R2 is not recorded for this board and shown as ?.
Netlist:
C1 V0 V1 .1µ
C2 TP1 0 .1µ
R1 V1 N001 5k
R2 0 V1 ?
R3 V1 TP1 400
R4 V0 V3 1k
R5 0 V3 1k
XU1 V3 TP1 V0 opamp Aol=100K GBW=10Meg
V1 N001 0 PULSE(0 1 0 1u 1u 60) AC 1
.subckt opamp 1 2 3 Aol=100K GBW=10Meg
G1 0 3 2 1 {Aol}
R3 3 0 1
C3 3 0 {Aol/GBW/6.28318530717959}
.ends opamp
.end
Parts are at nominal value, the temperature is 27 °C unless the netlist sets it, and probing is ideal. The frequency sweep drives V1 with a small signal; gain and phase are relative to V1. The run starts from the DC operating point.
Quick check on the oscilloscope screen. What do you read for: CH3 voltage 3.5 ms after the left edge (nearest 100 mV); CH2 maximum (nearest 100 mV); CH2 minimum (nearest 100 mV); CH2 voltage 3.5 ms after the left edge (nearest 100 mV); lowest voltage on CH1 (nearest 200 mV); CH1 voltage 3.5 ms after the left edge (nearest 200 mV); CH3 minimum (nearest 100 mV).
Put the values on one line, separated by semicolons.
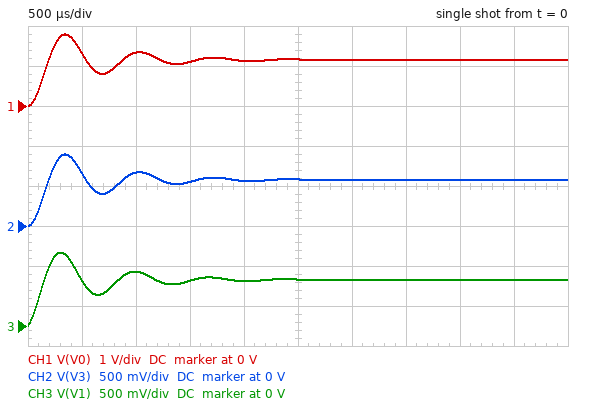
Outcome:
600 mV; 900 mV; 0 V; 600 mV; 0 V; 1.2 V; 0 V
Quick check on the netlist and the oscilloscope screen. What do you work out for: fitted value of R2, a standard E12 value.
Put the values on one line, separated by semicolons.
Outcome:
6.8 kΩ
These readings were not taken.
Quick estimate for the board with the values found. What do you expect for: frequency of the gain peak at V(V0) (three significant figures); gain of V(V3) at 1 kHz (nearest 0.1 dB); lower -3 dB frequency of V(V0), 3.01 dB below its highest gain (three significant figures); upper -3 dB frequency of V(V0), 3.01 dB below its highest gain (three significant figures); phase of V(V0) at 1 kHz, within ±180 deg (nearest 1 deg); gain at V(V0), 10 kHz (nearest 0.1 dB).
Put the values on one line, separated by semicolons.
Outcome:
1.43 kHz; -0.3 dB; 1.11 kHz; 1.69 kHz; -25 deg; -31.8 dB
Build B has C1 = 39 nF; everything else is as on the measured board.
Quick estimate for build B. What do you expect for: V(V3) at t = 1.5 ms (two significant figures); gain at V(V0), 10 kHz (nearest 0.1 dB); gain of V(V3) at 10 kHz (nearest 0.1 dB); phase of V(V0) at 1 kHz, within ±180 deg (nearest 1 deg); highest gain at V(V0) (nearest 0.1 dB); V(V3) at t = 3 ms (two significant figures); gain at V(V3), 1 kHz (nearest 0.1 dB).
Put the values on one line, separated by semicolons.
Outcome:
580 mV; -25.4 dB; -31.5 dB; -59 deg; 1.2 dB; 580 mV; -8.8 dB
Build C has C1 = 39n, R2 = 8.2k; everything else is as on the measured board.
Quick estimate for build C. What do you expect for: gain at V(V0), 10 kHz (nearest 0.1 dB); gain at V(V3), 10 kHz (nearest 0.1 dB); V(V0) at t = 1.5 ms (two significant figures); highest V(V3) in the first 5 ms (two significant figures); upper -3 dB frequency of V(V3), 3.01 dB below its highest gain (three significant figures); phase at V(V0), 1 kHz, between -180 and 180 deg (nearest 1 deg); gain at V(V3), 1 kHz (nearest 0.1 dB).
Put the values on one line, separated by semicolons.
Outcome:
-25.4 dB; -31.4 dB; 1.2 V; 620 mV; 763 Hz; -61 deg; -8.5 dB
